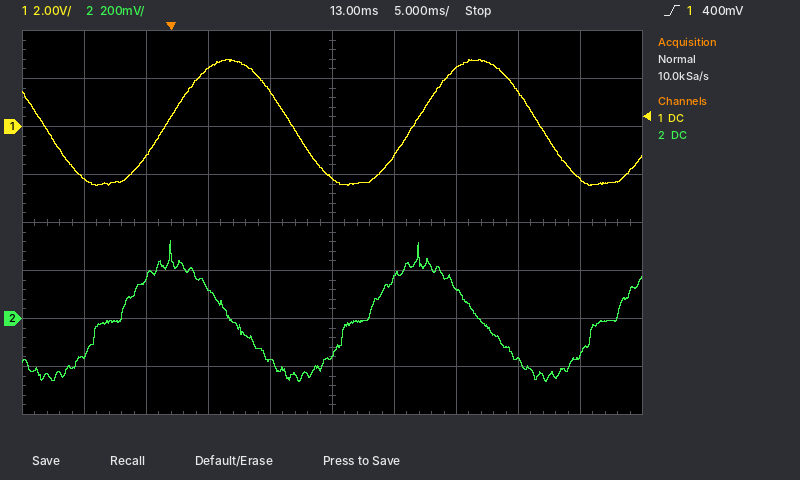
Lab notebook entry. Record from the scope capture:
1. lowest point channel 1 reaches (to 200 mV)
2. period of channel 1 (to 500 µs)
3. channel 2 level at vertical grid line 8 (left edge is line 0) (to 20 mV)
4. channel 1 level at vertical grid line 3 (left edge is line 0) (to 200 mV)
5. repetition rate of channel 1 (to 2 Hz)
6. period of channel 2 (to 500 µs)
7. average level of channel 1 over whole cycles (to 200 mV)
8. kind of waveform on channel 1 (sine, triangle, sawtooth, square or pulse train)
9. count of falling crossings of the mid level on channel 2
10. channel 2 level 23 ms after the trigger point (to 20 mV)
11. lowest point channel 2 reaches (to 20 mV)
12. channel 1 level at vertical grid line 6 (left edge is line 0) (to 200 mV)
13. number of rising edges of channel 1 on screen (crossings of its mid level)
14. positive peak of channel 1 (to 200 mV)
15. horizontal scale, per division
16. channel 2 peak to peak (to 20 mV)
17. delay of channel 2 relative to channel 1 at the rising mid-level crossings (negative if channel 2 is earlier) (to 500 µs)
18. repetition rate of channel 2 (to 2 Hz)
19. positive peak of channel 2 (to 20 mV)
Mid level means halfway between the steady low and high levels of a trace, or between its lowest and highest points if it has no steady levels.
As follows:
-2.4 V
20.0 ms
-180 mV
2.4 V
50 Hz
20.0 ms
200 mV
sine
2
120 mV
-260 mV
-1.2 V
2
2.8 V
5 ms
580 mV
-3.5 ms
50 Hz
320 mV
